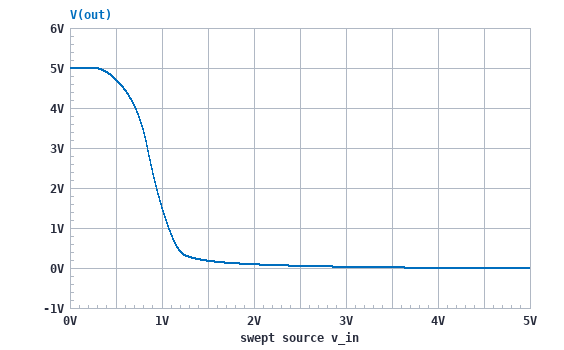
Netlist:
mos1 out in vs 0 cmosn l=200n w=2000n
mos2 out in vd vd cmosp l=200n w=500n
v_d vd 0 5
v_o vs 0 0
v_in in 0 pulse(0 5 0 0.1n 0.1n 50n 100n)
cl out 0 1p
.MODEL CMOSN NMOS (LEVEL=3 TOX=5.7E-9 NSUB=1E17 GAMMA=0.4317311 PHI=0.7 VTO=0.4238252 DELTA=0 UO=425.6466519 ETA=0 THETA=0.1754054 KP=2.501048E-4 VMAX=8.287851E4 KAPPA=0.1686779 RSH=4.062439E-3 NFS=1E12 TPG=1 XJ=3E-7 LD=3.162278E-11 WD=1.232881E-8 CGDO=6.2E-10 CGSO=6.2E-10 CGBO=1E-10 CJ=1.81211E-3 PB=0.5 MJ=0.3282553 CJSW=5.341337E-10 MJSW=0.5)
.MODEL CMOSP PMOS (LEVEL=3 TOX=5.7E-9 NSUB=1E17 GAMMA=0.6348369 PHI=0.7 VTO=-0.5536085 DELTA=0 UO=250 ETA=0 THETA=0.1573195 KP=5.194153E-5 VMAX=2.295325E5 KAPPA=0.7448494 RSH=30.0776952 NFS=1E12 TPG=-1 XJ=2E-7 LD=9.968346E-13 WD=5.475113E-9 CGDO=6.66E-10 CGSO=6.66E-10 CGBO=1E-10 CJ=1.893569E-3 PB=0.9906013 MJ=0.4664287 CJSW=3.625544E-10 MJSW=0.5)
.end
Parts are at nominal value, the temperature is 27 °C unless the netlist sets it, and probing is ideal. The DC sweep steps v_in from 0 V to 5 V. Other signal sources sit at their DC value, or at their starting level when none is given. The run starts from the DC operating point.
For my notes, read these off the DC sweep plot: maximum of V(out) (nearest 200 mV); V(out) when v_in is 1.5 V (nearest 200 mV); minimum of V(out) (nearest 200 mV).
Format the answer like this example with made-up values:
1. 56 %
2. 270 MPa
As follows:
1. 5.0 V
2. 200 mV
3. 0 V
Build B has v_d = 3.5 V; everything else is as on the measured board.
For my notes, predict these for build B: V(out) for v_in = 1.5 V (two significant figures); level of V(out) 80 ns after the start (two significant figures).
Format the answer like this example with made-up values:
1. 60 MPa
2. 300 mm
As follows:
1. 49 mV
2. 3.5 V
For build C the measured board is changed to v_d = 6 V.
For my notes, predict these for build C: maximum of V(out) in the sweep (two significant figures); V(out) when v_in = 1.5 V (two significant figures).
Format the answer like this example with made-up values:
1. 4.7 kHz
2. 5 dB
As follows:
1. 6.0 V
2. 420 mV
